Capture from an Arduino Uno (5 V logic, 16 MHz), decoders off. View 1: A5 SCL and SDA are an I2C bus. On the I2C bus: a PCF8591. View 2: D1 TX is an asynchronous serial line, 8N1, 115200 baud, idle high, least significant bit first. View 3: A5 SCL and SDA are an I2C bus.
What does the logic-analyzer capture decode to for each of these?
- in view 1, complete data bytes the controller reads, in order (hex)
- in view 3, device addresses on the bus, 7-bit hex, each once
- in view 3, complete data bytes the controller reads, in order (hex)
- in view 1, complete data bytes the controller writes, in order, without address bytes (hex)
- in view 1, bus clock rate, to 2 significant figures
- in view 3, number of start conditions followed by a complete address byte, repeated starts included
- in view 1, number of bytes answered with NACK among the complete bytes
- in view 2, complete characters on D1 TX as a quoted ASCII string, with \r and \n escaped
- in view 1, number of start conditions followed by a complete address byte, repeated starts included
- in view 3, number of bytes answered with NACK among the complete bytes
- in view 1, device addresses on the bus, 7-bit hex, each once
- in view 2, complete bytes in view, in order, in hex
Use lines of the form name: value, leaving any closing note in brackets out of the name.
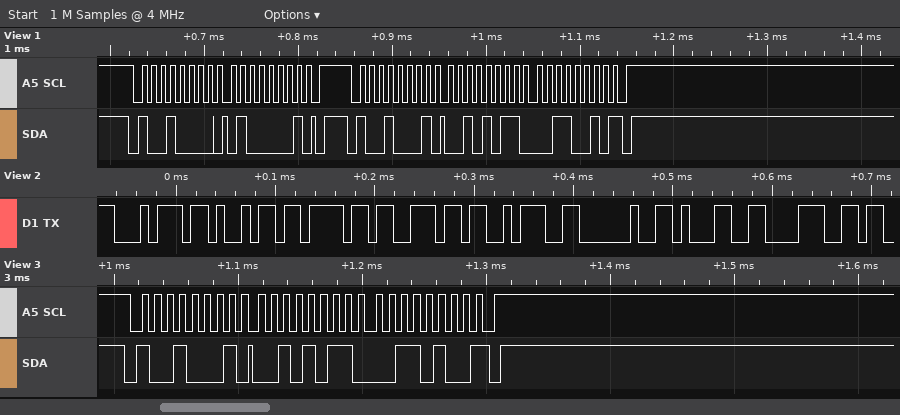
in view 1, complete data bytes the controller reads, in order: 2B 32
in view 3, device addresses on the bus, 7-bit hex, each once: 0x48
in view 3, complete data bytes the controller reads, in order: 2B 34
in view 1, complete data bytes the controller writes, in order, without address bytes: 41
in view 1, bus clock rate, to 2 significant figures: 100 kHz
in view 3, number of start conditions followed by a complete address byte, repeated starts included: 1
in view 1, number of bytes answered with NACK among the complete bytes: 1
in view 2, complete characters on D1 TX as a quoted ASCII string, with \r and \n escaped: "tion: 18"
in view 1, number of start conditions followed by a complete address byte, repeated starts included: 2
in view 3, number of bytes answered with NACK among the complete bytes: 1
in view 1, device addresses on the bus, 7-bit hex, each once: 0x48
in view 2, complete bytes in view, in order, in hex: 0x74 0x69 0x6F 0x6E 0x3A 0x20 0x31 0x38
